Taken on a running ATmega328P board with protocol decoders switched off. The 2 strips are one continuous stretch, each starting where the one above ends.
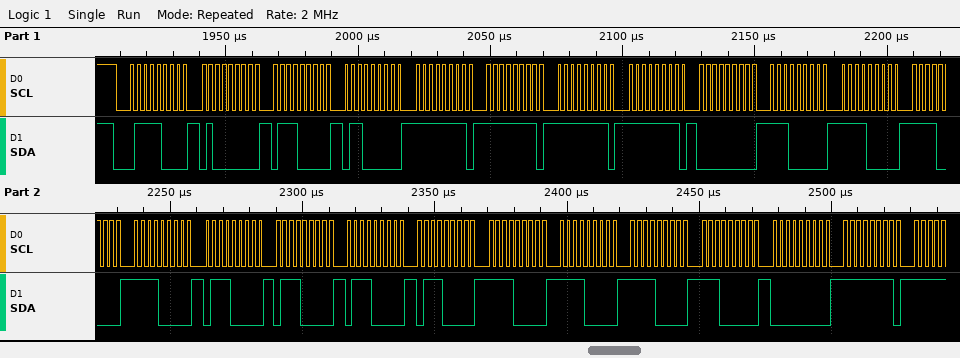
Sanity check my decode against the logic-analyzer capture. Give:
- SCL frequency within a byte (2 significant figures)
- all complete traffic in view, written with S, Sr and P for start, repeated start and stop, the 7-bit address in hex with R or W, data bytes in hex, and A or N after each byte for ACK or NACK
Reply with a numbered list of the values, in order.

1. 400 kHz
2. S 3CW A 40 A 70 A 60 A FF A FF A FF A FF A 00 A E0 A F0 A F0 A F0 A 70 A 70 A 70 A 70 A F0 A F0 A F0 A E0 A 00 A FF A
